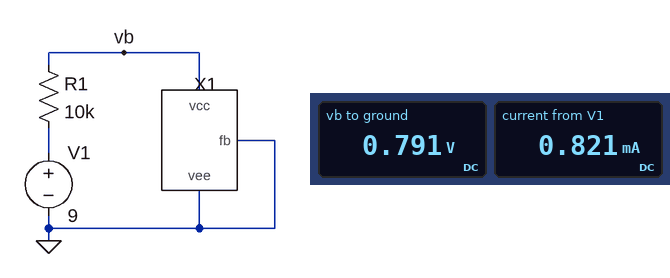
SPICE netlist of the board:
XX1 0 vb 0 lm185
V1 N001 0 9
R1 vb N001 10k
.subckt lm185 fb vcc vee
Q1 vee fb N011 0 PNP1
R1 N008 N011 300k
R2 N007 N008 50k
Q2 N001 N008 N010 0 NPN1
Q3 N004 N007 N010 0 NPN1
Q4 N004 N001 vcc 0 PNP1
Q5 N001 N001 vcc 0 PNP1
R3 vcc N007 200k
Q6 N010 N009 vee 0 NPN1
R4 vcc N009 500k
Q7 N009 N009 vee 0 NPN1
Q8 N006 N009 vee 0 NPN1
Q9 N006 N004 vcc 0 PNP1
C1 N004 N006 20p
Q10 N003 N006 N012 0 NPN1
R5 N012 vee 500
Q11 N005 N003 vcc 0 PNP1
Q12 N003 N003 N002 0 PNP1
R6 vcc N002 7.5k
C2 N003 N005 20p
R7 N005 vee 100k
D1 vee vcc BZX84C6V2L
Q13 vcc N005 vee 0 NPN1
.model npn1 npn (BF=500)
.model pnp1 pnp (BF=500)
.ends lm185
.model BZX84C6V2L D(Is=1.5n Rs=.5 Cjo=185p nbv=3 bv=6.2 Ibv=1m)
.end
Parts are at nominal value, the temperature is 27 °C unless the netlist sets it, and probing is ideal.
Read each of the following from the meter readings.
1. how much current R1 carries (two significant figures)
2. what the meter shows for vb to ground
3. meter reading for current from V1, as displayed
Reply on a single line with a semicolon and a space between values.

820 µA; 0.791 V; 0.821 mA
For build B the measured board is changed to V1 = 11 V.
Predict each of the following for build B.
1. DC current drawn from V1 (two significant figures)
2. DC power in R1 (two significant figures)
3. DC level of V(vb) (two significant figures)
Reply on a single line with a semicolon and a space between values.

1.0 mA; 10 mW; 800 mV
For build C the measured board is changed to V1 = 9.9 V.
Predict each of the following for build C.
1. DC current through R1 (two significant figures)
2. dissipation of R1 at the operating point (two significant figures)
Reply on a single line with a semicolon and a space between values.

910 µA; 8.3 mW
